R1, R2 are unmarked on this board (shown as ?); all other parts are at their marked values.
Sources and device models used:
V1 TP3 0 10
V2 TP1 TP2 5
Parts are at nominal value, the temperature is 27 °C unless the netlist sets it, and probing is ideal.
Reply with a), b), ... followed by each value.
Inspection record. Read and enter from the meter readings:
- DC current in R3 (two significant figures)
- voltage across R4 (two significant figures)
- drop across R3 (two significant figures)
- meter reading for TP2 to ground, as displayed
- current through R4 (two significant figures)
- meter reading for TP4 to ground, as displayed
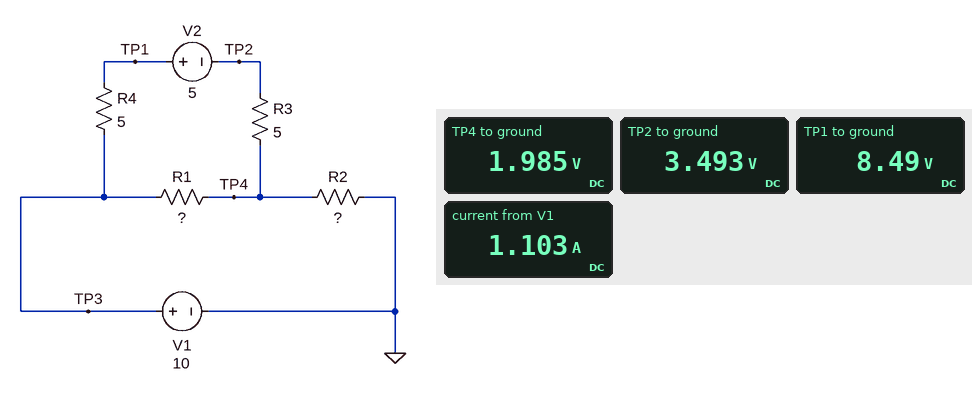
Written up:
a) 300 mA
b) 1.5 V
c) 1.5 V
d) 3.493 V
e) 300 mA
f) 1.985 V
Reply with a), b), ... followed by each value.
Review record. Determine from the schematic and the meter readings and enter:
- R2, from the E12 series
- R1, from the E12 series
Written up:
a) 1.8 Ω
b) 10 Ω
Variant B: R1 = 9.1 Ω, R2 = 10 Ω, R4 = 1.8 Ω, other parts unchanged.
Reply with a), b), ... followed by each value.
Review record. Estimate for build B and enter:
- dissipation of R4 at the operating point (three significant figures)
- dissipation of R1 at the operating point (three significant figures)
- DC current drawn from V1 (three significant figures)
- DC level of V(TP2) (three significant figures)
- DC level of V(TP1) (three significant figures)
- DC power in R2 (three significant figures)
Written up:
a) 747 µW
b) 2.60 W
c) 514 mA
d) 5.04 V
e) 10.0 V
f) 2.64 W
